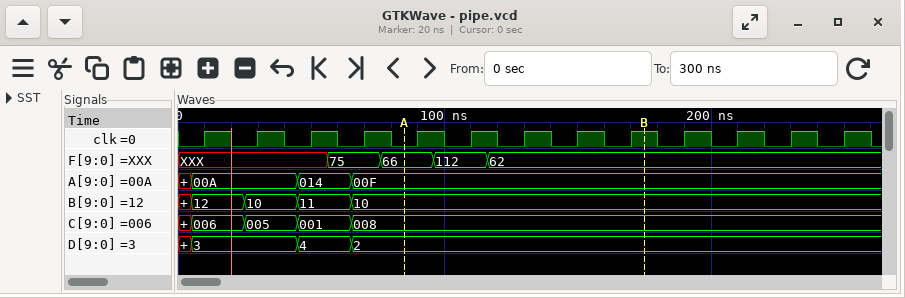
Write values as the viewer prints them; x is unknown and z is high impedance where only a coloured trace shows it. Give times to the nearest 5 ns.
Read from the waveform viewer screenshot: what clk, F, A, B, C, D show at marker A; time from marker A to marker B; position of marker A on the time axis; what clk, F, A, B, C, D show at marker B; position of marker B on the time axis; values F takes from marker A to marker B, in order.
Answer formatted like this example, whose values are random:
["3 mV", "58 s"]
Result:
["clk=0, F=66, A=00F, B=10, C=008, D=2", "90 ns", "85 ns", "clk=1, F=62, A=00F, B=10, C=008, D=2", "175 ns", "66, 112, 62"]
